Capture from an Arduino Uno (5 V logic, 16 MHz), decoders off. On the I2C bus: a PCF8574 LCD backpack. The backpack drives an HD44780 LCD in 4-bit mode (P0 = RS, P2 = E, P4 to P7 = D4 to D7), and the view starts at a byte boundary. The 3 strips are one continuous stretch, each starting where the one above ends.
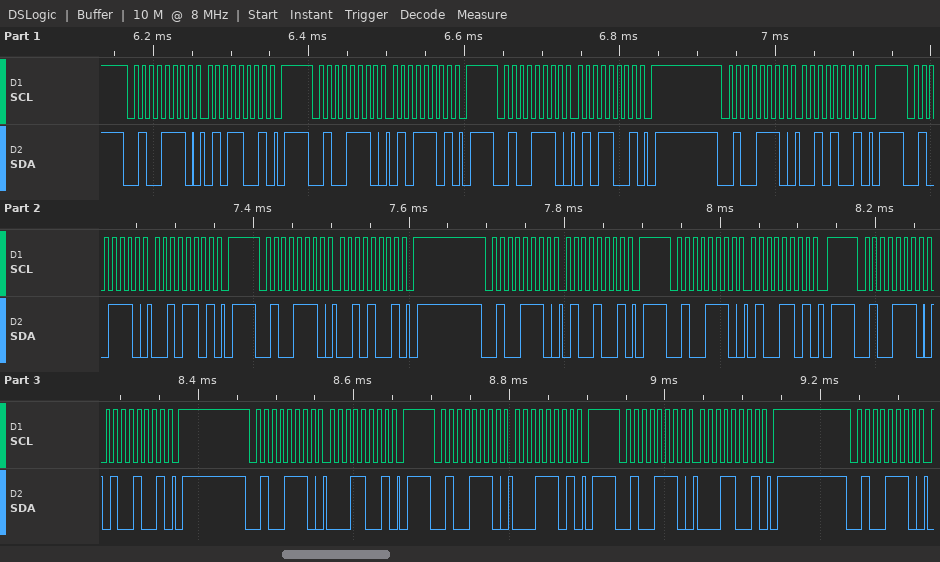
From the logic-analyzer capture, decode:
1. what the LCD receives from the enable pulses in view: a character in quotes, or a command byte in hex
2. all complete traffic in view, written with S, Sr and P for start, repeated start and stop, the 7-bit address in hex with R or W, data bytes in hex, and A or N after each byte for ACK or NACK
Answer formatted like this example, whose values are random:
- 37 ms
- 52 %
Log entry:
- 'R' 'A'
- S 27W A 59 A P S 27W A 5D A P S 27W A 59 A P S 27W A 29 A P S 27W A 2D A P S 27W A 29 A P S 27W A 49 A P S 27W A 4D A P S 27W A 49 A P S 27W A 19 A P S 27W A 1D A P S 27W A 19 A P S 27W A
